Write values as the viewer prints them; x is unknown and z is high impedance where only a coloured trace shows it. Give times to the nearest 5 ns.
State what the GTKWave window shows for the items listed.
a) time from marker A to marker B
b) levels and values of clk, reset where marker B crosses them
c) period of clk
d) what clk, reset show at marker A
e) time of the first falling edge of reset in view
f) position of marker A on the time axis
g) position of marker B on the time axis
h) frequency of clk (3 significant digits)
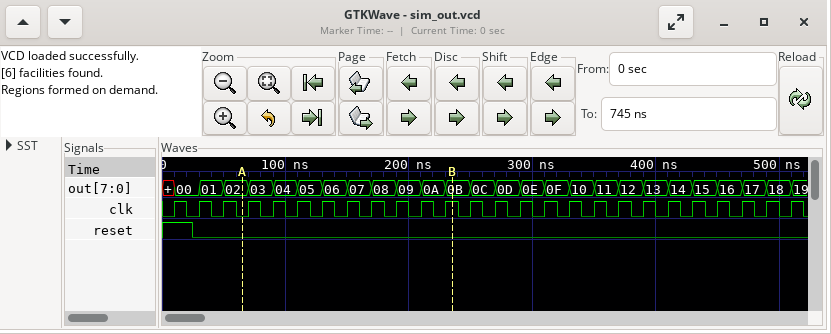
170 ns
clk=1, reset=0
20 ns
clk=0, reset=0
25 ns
65 ns
235 ns
50.0 MHz
